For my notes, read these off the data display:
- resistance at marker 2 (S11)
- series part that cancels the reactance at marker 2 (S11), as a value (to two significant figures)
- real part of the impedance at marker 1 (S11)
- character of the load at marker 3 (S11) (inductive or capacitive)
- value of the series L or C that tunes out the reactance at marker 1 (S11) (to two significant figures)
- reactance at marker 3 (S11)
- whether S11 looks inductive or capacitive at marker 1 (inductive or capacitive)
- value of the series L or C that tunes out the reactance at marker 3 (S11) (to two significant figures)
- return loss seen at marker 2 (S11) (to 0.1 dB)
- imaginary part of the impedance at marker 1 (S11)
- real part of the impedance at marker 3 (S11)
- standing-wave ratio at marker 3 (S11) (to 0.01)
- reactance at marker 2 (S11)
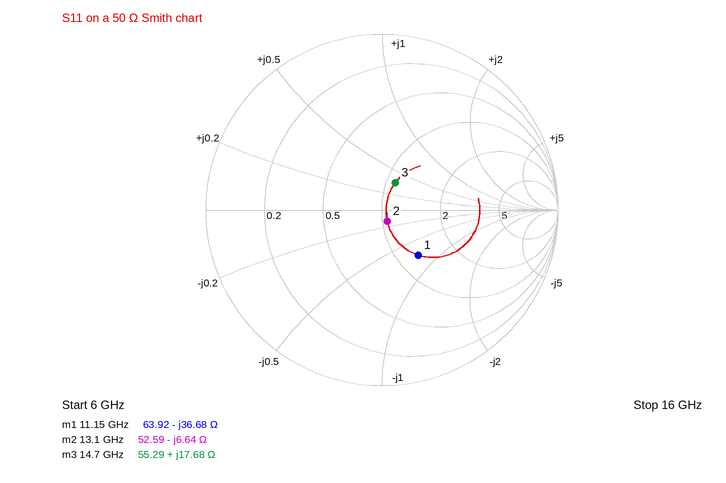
52.59 Ω
81 pH
63.92 Ω
inductive
520 pH
+17.68 Ω
capacitive
610 fF
23.2 dB
-36.68 Ω
55.29 Ω
1.42
-6.64 Ω
